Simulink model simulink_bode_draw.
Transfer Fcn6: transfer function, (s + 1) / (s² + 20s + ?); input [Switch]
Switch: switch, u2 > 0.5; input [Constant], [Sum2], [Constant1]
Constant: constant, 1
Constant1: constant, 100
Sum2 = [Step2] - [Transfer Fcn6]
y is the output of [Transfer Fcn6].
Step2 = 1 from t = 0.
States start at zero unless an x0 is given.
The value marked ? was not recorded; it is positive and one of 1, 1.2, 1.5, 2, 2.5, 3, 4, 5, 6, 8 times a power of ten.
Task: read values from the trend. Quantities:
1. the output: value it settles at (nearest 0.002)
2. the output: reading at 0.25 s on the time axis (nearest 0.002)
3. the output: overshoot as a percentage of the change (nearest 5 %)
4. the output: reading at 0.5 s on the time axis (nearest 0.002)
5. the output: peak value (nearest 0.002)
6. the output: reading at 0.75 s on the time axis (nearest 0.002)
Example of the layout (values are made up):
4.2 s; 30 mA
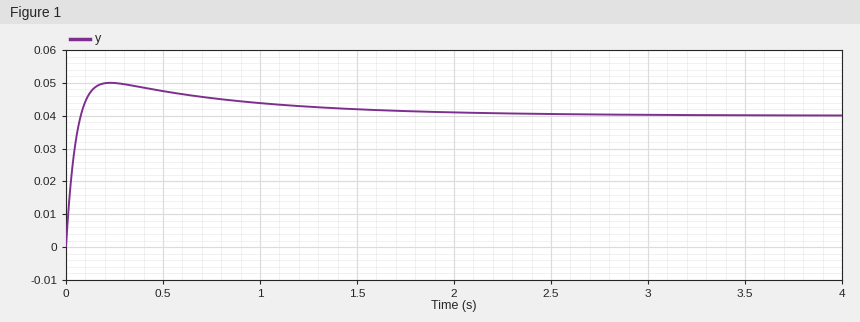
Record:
0.040; 0.050; 25 %; 0.048; 0.050; 0.046
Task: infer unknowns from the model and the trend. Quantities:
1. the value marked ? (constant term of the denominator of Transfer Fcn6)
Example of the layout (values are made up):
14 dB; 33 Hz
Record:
25
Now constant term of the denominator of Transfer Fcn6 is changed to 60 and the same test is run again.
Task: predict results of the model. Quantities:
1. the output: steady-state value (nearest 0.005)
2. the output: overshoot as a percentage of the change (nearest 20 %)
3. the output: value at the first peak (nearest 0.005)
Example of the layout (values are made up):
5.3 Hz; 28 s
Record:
0.015; 160 %; 0.045
